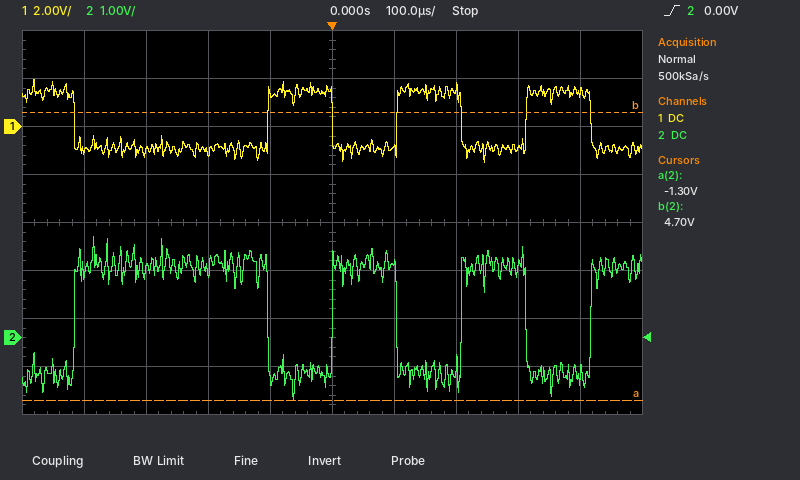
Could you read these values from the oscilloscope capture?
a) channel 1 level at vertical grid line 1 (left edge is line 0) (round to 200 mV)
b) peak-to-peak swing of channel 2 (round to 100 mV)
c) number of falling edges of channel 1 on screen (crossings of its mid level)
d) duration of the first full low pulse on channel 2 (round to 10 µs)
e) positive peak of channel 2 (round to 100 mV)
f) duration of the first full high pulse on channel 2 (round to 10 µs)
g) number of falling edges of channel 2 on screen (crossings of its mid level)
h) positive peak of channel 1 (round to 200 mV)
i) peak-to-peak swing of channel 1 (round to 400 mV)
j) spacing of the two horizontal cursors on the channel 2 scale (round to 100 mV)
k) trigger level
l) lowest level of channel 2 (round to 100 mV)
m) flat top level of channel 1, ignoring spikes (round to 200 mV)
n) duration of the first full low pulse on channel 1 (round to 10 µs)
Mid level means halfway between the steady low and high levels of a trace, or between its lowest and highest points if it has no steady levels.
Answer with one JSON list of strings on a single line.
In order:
["-1.0 V", "3.4 V", "4", "100 µs", "2.1 V", "310 µs", "3", "2.0 V", "3.6 V", "6.0 V", "0.00 V", "-1.3 V", "1.4 V", "310 µs"]
